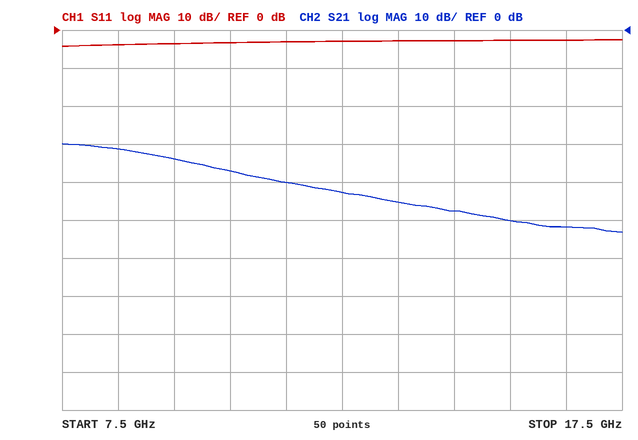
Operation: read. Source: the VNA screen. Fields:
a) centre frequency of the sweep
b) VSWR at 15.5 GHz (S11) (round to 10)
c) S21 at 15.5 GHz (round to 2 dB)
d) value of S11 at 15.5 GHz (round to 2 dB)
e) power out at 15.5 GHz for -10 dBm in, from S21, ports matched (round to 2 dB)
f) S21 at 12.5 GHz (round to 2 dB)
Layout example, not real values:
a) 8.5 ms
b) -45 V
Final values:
a) 12.5 GHz
b) 10
c) -50 dB
d) -2 dB
e) -60 dBm
f) -42 dB
